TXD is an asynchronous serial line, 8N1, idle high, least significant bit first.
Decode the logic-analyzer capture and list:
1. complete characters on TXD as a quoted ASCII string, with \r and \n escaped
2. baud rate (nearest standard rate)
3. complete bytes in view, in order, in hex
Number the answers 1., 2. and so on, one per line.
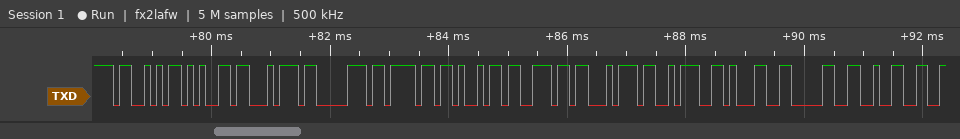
1. "Setpoint:102"
2. 9600 baud
3. 53 65 74 70 6F 69 6E 74 3A 31 30 32
